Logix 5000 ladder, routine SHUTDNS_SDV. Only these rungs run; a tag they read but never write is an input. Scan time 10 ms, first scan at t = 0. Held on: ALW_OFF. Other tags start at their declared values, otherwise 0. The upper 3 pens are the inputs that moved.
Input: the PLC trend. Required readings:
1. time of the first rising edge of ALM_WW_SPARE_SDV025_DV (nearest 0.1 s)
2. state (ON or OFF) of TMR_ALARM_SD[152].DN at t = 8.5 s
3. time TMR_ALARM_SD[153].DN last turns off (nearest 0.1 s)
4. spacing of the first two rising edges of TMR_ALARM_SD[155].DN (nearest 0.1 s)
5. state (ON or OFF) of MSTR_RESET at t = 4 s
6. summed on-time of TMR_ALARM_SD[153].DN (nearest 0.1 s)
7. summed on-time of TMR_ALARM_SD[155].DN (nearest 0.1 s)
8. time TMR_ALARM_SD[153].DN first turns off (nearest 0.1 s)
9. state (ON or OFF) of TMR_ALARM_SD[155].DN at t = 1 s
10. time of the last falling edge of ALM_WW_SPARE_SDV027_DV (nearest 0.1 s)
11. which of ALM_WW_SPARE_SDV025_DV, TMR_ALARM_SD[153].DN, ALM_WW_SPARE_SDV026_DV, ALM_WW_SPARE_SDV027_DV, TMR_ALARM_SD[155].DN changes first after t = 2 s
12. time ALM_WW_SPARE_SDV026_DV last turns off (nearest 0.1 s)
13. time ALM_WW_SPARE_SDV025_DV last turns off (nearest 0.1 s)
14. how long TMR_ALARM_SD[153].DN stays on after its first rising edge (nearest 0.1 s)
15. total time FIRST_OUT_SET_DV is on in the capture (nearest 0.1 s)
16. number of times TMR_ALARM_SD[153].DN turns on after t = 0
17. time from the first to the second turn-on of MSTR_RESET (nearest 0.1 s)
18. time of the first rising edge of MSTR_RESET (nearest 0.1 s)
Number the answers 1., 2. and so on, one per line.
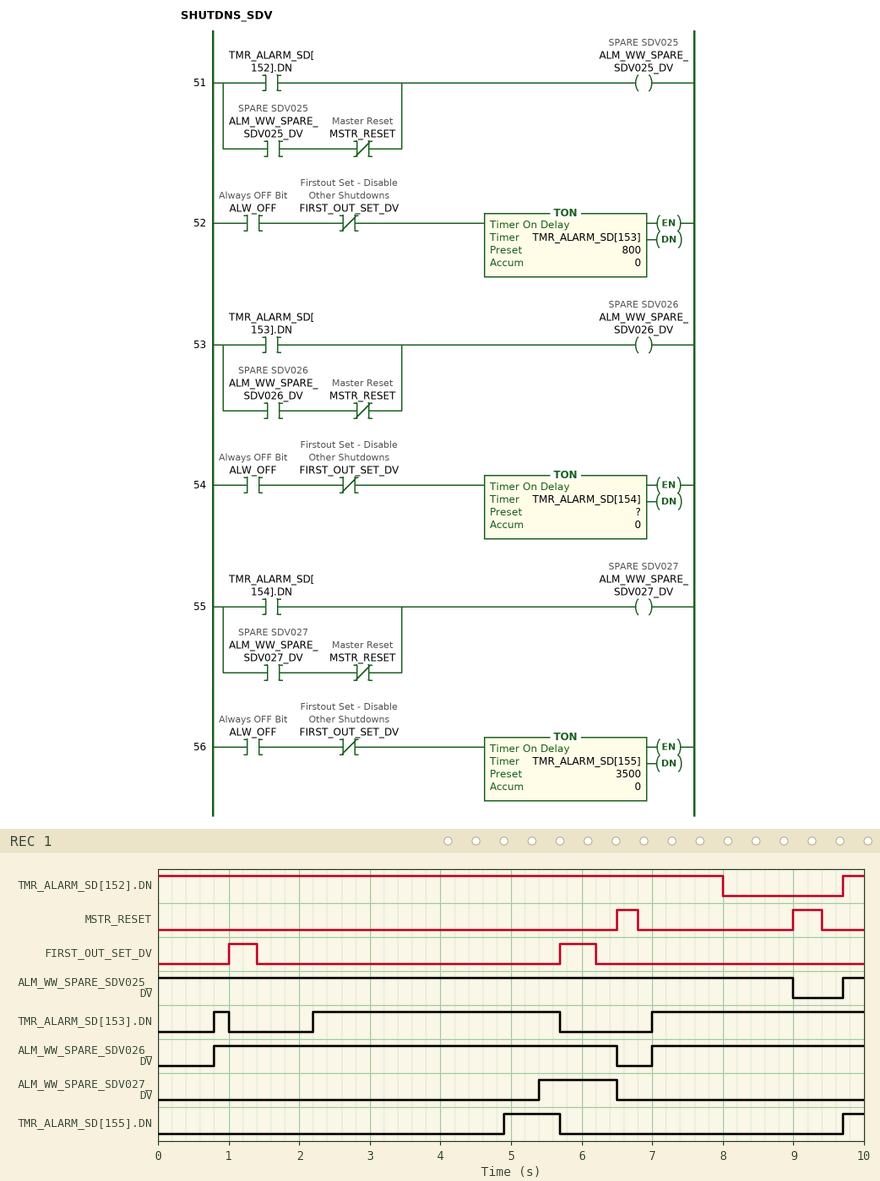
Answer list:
1. 9.7 s
2. OFF
3. 5.7 s
4. 4.8 s
5. OFF
6. 6.7 s
7. 1.1 s
8. 1.0 s
9. OFF
10. 6.5 s
11. TMR_ALARM_SD[153].DN
12. 6.5 s
13. 9.0 s
14. 0.2 s
15. 0.9 s
16. 3
17. 2.5 s
18. 6.5 s
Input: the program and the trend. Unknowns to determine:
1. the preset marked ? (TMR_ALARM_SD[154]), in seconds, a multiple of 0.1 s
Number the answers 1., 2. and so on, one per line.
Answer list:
1. 4.0 s
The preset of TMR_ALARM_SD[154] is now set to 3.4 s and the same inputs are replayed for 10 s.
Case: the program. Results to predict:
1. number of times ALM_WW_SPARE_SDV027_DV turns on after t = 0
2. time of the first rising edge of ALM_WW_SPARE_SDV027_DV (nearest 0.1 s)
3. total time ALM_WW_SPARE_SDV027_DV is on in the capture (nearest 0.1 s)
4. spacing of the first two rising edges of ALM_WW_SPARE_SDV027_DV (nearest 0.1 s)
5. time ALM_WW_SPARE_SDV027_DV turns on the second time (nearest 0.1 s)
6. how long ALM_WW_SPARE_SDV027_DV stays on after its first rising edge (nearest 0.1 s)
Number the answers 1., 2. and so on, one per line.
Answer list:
1. 2
2. 4.8 s
3. 2.1 s
4. 4.8 s
5. 9.6 s
6. 1.7 s
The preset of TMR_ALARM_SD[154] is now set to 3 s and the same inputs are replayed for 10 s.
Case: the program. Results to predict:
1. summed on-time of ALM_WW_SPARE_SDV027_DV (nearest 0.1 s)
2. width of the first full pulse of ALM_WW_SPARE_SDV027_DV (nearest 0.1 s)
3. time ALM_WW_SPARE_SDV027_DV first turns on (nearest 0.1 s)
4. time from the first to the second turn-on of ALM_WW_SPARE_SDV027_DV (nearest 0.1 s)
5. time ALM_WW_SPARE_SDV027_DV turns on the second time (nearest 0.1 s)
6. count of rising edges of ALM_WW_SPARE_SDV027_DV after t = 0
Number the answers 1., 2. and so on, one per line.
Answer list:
1. 2.9 s
2. 2.1 s
3. 4.4 s
4. 4.8 s
5. 9.2 s
6. 2
